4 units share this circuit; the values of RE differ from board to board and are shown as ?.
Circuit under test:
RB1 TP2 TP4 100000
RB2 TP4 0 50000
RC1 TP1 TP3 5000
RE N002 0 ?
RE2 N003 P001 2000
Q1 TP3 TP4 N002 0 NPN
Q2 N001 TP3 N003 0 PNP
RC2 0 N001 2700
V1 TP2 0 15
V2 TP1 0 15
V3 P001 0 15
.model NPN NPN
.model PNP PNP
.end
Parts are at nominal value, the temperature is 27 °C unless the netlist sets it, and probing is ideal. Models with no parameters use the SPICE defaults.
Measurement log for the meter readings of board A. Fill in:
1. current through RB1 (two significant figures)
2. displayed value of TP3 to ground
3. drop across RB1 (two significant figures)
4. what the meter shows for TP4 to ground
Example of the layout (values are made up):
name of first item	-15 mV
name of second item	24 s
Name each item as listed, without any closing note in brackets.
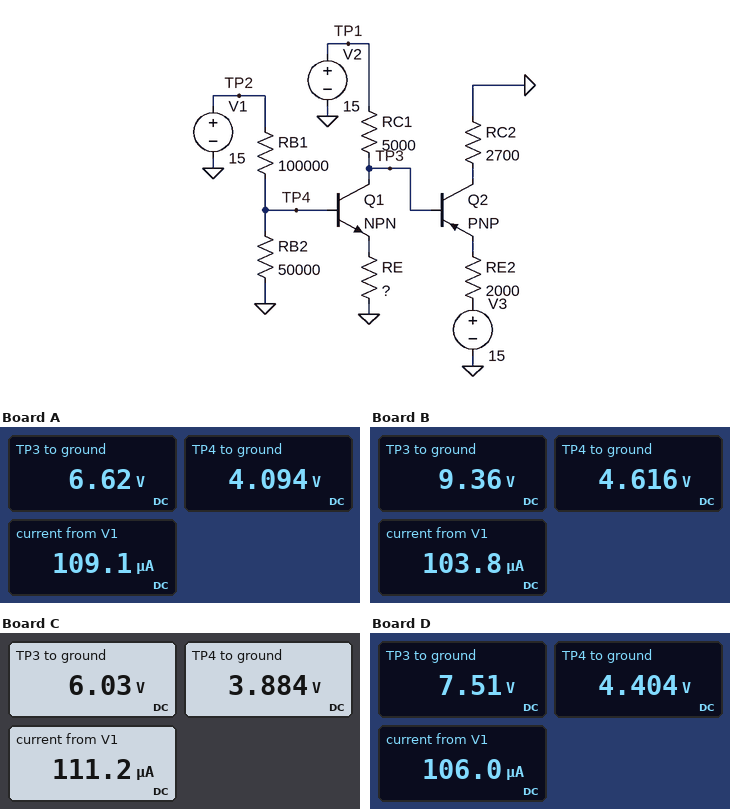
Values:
current through RB1	110 µA
displayed value of TP3 to ground	6.62 V
drop across RB1	11 V
what the meter shows for TP4 to ground	4.094 V
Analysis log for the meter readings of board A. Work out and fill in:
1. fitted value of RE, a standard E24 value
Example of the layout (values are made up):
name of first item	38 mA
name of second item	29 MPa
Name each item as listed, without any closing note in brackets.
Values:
fitted value of RE, a standard E24 value	1.2 kΩ
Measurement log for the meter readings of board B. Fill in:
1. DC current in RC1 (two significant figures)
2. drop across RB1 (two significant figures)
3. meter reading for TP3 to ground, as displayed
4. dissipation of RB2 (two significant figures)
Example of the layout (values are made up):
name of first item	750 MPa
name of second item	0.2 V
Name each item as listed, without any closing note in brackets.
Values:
DC current in RC1	1.1 mA
drop across RB1	10 V
meter reading for TP3 to ground, as displayed	9.36 V
dissipation of RB2	430 µW
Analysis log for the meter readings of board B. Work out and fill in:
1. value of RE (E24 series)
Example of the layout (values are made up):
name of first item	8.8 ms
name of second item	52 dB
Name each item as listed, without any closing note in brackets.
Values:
value of RE	3.3 kΩ
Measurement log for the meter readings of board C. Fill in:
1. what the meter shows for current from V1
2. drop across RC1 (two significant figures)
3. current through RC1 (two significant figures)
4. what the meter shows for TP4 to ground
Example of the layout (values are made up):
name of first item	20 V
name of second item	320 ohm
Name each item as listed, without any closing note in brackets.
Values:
what the meter shows for current from V1	111.2 µA
drop across RC1	9.0 V
current through RC1	1.8 mA
what the meter shows for TP4 to ground	3.884 V
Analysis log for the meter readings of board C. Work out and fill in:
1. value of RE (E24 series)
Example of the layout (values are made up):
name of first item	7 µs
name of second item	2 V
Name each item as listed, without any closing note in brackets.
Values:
value of RE	910 Ω
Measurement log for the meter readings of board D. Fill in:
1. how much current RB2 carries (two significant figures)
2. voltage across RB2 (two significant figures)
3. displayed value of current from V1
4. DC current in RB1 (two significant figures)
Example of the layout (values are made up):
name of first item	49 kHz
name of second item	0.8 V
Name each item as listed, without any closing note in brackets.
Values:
how much current RB2 carries	88 µA
voltage across RB2	4.4 V
displayed value of current from V1	106.0 µA
DC current in RB1	110 µA
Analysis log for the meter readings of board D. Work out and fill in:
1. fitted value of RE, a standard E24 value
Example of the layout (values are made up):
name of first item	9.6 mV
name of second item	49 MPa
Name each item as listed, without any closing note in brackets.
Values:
fitted value of RE, a standard E24 value	2 kΩ
